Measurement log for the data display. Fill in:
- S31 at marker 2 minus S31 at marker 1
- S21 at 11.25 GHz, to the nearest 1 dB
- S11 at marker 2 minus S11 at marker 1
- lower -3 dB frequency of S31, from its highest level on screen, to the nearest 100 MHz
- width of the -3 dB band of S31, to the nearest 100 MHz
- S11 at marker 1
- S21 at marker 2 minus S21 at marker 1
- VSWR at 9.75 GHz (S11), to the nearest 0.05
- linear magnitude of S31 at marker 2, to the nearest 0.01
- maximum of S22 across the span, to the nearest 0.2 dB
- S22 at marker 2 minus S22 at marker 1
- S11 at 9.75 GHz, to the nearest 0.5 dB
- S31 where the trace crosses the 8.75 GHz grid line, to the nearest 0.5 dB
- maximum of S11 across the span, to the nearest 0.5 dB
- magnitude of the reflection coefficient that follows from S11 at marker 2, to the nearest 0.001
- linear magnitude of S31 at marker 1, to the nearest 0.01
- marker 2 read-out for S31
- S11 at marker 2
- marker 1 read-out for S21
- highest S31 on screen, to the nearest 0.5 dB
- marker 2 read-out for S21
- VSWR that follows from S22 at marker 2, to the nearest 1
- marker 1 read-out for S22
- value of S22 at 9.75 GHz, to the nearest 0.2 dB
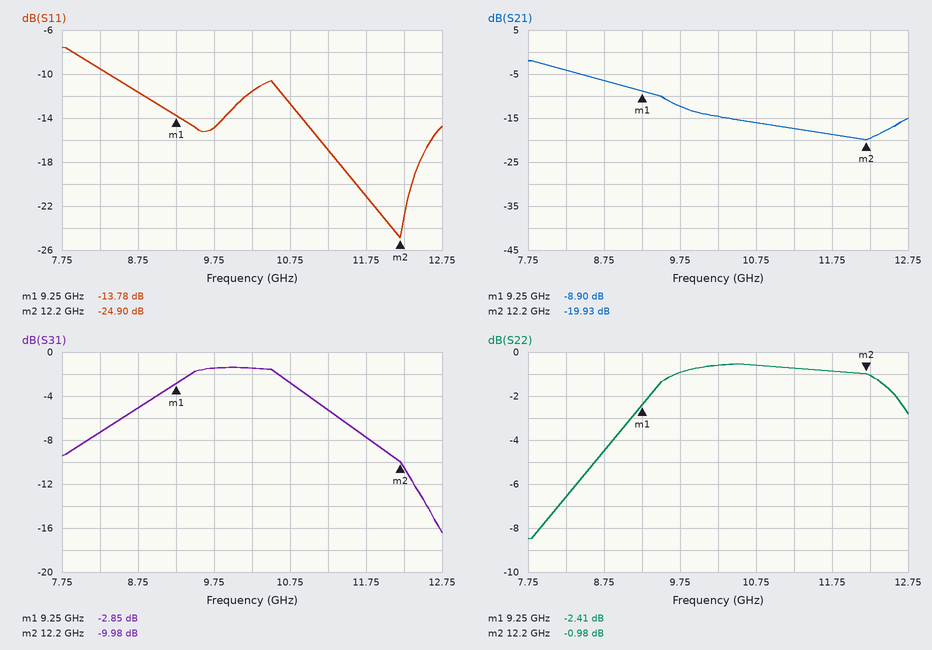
-7.13 dB
-17 dB
-11.12 dB
8.9 GHz
2.2 GHz
-13.78 dB
-11.03 dB
1.45
0.32
-0.6 dB
1.43 dB
-15.0 dB
-5.0 dB
-7.5 dB
0.057
0.72
-9.98 dB
-24.90 dB
-8.90 dB
-1.5 dB
-19.93 dB
18
-2.41 dB
-1.0 dB
